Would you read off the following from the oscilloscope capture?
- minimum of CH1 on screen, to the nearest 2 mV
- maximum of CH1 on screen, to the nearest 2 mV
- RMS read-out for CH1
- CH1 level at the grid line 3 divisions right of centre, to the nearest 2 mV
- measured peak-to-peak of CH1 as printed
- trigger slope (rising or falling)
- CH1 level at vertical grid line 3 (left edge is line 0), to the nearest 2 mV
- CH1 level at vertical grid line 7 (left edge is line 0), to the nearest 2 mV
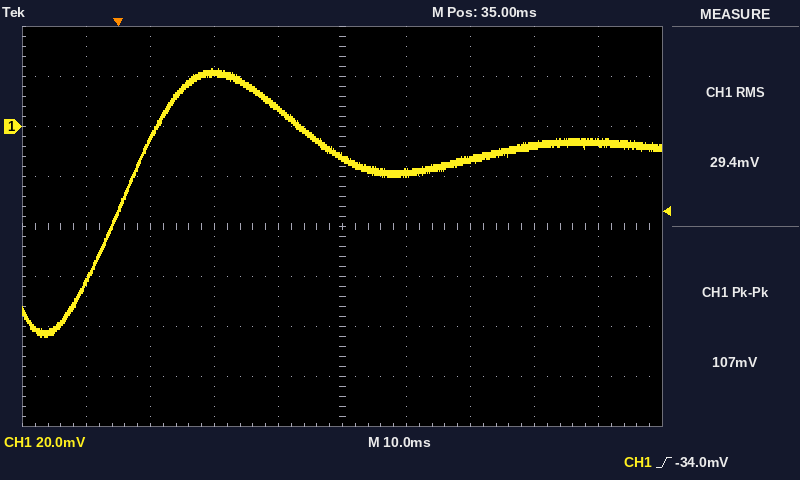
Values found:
-84 mV
24 mV
29.4 mV
-8 mV
107 mV
rising
22 mV
-14 mV
